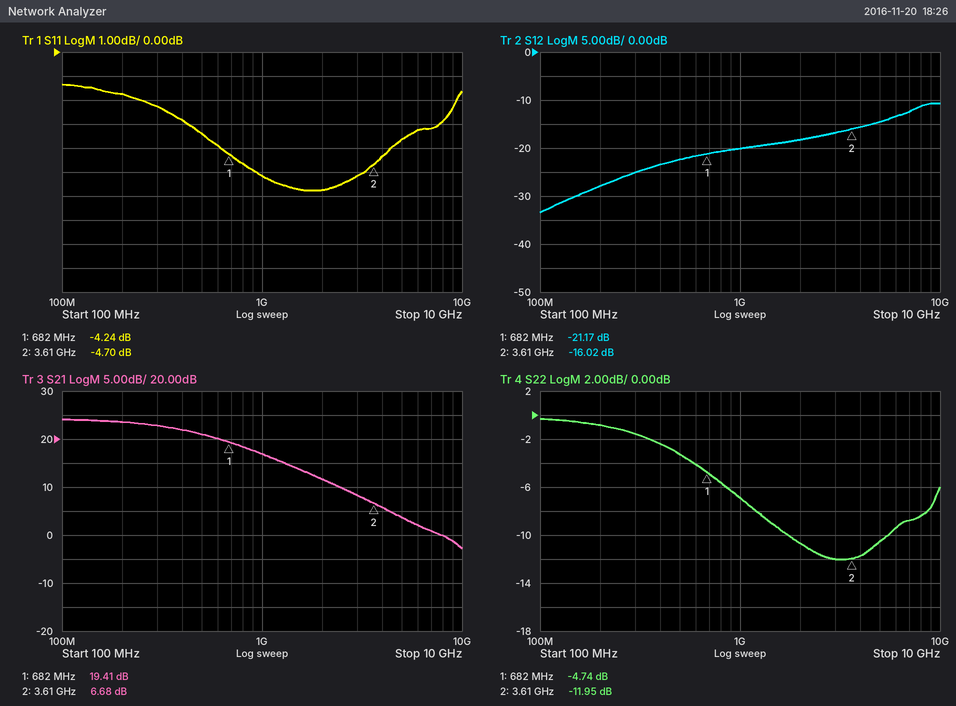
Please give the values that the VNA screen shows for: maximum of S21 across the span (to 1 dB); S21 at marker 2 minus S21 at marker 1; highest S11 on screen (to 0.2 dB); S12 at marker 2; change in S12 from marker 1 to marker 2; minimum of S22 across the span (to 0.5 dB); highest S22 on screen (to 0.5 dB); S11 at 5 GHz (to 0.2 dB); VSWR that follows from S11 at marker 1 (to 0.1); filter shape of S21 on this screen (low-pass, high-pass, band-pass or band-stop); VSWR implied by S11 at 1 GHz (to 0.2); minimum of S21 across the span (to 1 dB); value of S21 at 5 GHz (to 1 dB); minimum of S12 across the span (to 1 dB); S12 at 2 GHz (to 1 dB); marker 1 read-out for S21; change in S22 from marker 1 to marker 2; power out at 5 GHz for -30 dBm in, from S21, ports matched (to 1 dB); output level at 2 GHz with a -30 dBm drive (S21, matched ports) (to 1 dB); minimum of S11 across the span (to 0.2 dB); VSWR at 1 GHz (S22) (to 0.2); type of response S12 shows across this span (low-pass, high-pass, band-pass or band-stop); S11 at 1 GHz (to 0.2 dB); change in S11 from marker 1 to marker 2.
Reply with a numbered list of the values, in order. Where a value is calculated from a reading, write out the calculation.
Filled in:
1. 24 dB
2. 6.68 − (19.41) = -12.73 dB
3. -1.4 dB
4. -16.02 dB
5. -16.02 − (-21.17) = 5.15 dB
6. -12.0 dB
7. -0.5 dB
8. -3.6 dB
9. (1 + 0.6138)/(1 − 0.6138) ≈ 4.2
10. low-pass
11. |Γ| = 10^(-5.2/20) = 0.5495; VSWR = (1 + 0.5495)/(1 − 0.5495) ≈ 3.4
12. -3 dB
13. 4 dB
14. -33 dB
15. -18 dB
16. 19.41 dB
17. -11.95 − (-4.74) = -7.21 dB
18. -30 dBm + (4 dB) = -26 dBm
19. -30 dBm + (12 dB) = -18 dBm
20. -5.8 dB
21. |Γ| = 10^(-7/20) = 0.4467; VSWR = (1 + 0.4467)/(1 − 0.4467) ≈ 2.6
22. high-pass
23. -5.2 dB
24. -4.7 − (-4.24) = -0.46 dB
